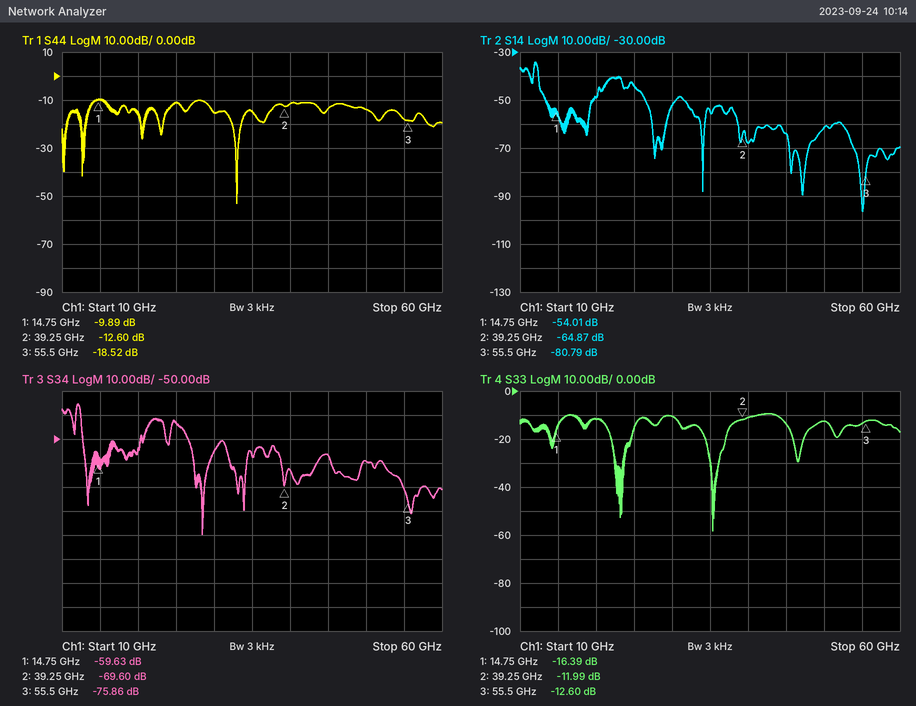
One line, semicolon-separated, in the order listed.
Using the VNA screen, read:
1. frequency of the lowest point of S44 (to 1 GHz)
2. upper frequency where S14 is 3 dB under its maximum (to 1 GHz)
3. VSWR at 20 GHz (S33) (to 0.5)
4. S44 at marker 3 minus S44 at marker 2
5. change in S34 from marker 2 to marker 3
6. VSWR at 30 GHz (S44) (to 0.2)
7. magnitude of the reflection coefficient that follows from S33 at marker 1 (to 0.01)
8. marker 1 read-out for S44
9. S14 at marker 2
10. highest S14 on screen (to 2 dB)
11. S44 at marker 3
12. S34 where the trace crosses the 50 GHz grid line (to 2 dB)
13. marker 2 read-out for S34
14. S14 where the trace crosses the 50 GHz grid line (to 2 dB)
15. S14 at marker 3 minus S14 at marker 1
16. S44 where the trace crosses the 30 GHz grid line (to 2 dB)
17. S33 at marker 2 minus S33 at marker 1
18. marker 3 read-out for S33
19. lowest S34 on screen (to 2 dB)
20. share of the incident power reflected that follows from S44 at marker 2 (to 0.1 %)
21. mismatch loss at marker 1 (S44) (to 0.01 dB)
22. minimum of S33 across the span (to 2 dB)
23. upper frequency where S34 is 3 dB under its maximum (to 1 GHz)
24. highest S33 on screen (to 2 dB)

33 GHz; 12 GHz; 1.5; -5.92 dB; -6.26 dB; 1.4; 0.15; -9.89 dB; -64.87 dB; -34 dB; -18.52 dB; -60 dB; -69.60 dB; -62 dB; -26.78 dB; -16 dB; 4.40 dB; -12.60 dB; -90 dB; 5.5 %; 0.47 dB; -58 dB; 12 GHz; -10 dB
